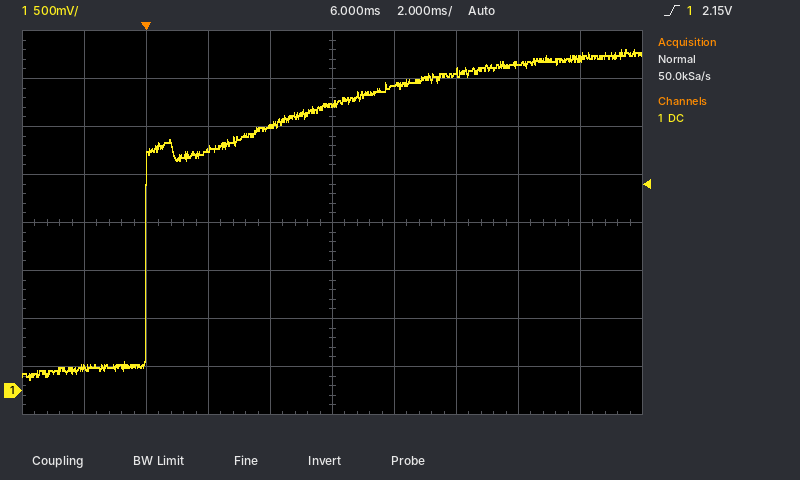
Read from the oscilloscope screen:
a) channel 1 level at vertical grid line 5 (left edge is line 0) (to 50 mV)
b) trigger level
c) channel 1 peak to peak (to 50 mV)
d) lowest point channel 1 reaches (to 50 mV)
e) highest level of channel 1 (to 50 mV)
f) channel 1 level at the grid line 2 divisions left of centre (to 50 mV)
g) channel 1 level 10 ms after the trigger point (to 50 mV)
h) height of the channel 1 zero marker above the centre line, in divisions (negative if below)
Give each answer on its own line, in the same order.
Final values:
3.00 V
2.15 V
3.45 V
100 mV
3.55 V
2.50 V
3.30 V
-3.5 div
